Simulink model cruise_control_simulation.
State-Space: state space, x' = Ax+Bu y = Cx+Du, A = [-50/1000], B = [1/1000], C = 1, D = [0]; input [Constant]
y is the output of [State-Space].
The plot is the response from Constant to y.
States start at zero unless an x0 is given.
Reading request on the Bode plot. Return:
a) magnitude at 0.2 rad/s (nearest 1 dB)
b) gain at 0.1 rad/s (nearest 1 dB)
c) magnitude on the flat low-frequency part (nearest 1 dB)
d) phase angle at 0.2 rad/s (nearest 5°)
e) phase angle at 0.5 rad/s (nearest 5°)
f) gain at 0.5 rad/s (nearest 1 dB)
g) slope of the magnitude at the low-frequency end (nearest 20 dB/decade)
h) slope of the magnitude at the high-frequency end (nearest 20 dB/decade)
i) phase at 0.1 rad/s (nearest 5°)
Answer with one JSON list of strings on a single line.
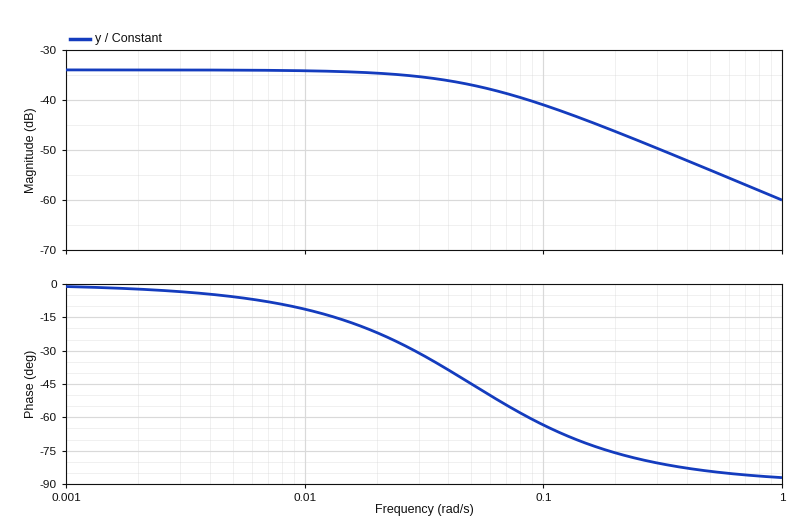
["-46 dB", "-41 dB", "-34 dB", "-75°", "-85°", "-54 dB", "0 dB/decade", "-20 dB/decade", "-65°"]
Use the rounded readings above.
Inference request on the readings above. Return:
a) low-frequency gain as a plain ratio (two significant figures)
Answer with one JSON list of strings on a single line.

["0.020"]
